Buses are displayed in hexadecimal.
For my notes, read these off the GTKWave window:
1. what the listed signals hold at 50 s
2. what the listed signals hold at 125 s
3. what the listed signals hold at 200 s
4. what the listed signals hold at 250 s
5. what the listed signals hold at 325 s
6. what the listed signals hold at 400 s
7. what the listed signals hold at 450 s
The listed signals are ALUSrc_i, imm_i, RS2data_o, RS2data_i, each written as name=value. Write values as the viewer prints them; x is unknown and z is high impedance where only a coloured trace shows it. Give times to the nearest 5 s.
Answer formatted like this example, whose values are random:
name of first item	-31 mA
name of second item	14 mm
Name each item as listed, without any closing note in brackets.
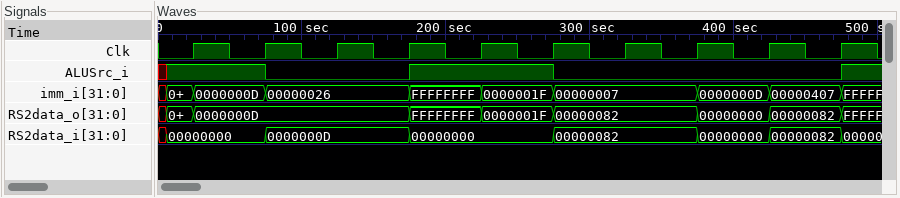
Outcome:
what the listed signals hold at 50 s	ALUSrc_i=1, imm_i=0000000D, RS2data_o=0000000D, RS2data_i=00000000
what the listed signals hold at 125 s	ALUSrc_i=0, imm_i=00000026, RS2data_o=0000000D, RS2data_i=0000000D
what the listed signals hold at 200 s	ALUSrc_i=1, imm_i=FFFFFFFF, RS2data_o=FFFFFFFF, RS2data_i=00000000
what the listed signals hold at 250 s	ALUSrc_i=1, imm_i=0000001F, RS2data_o=0000001F, RS2data_i=00000000
what the listed signals hold at 325 s	ALUSrc_i=0, imm_i=00000007, RS2data_o=00000082, RS2data_i=00000082
what the listed signals hold at 400 s	ALUSrc_i=0, imm_i=0000000D, RS2data_o=00000000, RS2data_i=00000000
what the listed signals hold at 450 s	ALUSrc_i=0, imm_i=00000407, RS2data_o=00000082, RS2data_i=00000082
